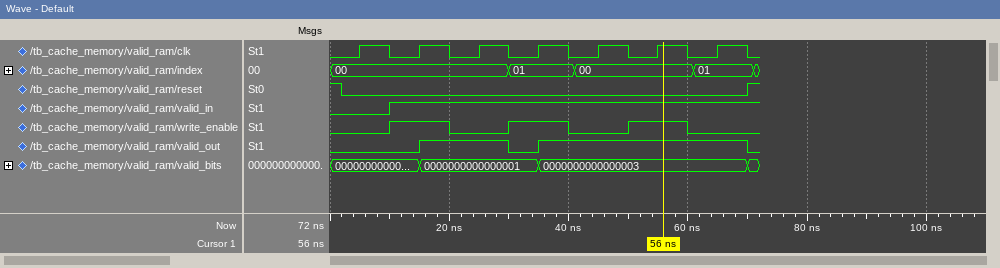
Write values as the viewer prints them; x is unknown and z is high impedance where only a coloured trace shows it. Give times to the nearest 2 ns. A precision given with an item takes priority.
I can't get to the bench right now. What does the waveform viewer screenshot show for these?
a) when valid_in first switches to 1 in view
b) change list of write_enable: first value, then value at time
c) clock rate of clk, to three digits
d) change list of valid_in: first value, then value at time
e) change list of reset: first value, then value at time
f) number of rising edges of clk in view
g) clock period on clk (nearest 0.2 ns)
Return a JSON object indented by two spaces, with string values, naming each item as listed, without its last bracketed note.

{
  "when valid_in first switches to 1 in view": "10 ns",
  "change list of write_enable: first value, then value at time": "0, 1 at 10 ns, 0 at 20 ns, 1 at 30 ns, 0 at 40 ns, 1 at 50 ns, 0 at 60 ns",
  "clock rate of clk, to three digits": "100 MHz",
  "change list of valid_in: first value, then value at time": "0, 1 at 10 ns",
  "change list of reset: first value, then value at time": "1, 0 at 2 ns, 1 at 70 ns",
  "number of rising edges of clk in view": "7",
  "clock period on clk": "10 ns"
}
